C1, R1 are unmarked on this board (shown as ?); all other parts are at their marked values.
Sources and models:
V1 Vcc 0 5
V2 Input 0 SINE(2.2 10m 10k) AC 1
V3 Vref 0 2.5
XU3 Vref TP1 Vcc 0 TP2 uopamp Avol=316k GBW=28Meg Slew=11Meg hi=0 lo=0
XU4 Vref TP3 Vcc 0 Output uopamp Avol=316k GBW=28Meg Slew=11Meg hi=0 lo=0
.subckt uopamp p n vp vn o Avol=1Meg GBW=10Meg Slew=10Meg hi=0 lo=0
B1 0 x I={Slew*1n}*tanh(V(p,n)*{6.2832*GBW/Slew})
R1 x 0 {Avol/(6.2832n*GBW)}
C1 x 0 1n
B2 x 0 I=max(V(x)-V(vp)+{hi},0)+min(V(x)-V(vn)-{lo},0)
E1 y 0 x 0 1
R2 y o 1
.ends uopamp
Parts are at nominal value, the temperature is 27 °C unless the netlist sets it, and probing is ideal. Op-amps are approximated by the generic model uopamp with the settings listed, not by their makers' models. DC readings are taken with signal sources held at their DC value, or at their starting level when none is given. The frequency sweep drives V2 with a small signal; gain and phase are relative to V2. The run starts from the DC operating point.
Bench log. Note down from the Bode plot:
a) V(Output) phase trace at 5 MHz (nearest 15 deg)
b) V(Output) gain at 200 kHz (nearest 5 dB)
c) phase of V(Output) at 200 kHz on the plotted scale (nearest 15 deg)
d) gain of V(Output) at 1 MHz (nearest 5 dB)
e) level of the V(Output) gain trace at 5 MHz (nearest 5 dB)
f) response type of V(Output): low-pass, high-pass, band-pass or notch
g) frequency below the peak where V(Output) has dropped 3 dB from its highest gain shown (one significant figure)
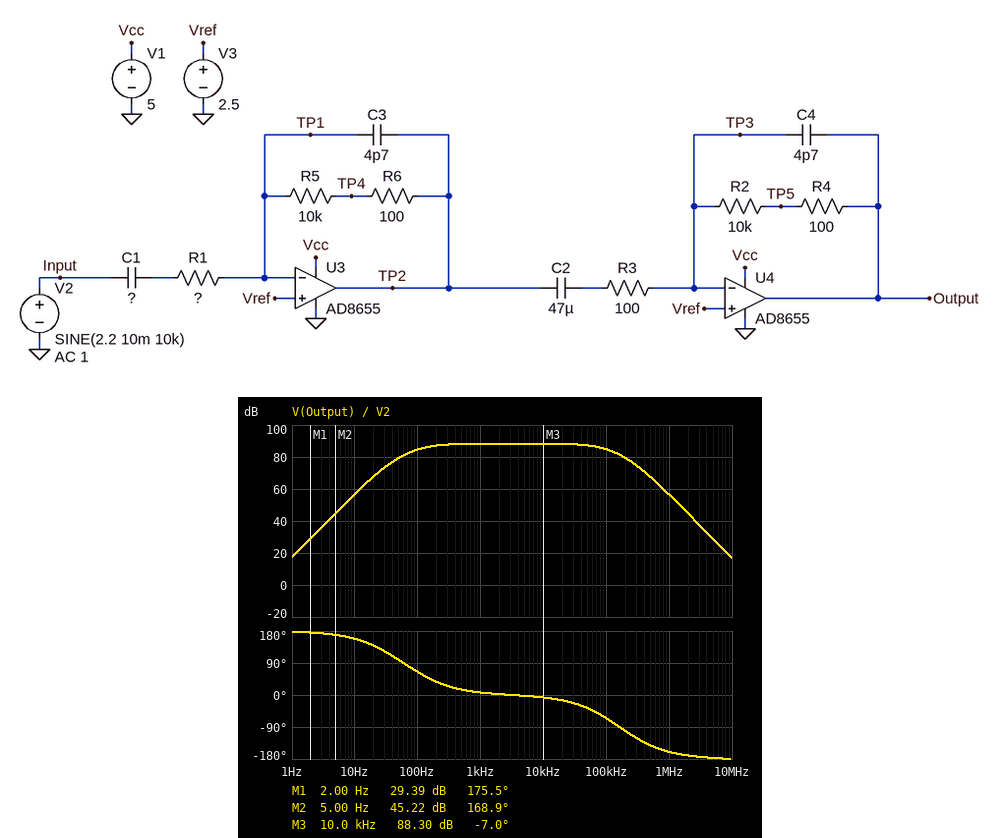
-180 deg
80 dB
-105 deg
55 dB
30 dB
band-pass
100 Hz
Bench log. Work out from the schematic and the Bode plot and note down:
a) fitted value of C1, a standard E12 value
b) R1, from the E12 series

39 µF
39 Ω
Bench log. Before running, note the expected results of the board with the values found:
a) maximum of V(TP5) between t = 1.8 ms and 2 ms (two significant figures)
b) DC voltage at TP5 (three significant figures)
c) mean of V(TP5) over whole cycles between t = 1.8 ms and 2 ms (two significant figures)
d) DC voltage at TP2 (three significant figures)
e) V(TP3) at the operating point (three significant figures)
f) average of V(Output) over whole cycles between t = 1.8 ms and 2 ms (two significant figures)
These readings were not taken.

5.0 V
2.50 V
2.5 V
2.50 V
2.50 V
2.5 V
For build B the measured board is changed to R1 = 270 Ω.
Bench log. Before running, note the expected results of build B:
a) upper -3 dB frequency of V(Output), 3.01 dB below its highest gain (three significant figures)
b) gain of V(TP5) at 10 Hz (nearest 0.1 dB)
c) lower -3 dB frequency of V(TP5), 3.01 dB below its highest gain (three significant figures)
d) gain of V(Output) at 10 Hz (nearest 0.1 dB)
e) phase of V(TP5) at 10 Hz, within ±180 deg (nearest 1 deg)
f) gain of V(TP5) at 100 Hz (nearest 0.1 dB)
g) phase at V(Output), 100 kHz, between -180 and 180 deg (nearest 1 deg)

221 kHz
55.3 dB
39.3 Hz
55.4 dB
130 deg
70.9 dB
-31 deg
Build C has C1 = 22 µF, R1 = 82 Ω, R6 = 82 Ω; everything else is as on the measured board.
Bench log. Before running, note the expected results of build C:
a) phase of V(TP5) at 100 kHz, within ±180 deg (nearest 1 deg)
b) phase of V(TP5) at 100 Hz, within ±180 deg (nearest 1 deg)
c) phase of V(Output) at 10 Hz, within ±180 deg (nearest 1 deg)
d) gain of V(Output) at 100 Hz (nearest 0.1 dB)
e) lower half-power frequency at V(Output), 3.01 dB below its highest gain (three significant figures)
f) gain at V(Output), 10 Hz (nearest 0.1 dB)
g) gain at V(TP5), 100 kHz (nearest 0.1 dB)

-47 deg
60 deg
157 deg
78.9 dB
99.1 Hz
52.0 dB
80.3 dB
